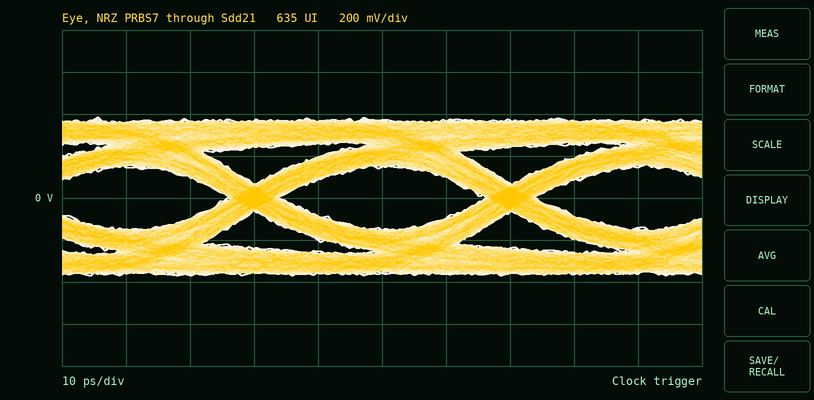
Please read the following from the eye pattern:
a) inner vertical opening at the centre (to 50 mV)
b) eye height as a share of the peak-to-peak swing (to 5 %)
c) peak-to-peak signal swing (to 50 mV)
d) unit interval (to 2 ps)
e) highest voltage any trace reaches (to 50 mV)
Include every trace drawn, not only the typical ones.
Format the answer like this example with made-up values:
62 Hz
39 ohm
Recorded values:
300 mV
40 %
750 mV
40 ps
400 mV
